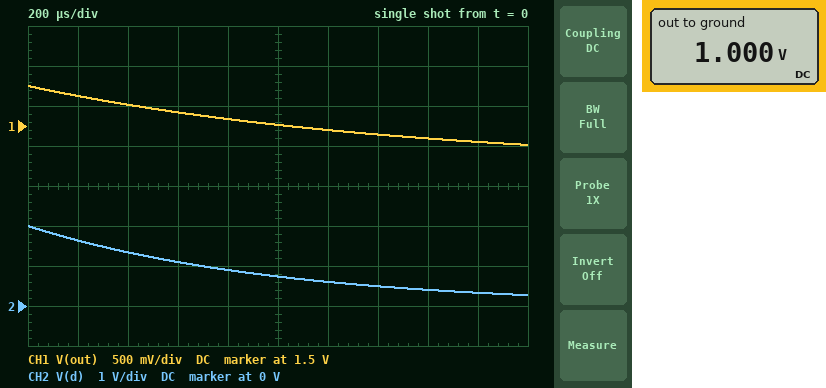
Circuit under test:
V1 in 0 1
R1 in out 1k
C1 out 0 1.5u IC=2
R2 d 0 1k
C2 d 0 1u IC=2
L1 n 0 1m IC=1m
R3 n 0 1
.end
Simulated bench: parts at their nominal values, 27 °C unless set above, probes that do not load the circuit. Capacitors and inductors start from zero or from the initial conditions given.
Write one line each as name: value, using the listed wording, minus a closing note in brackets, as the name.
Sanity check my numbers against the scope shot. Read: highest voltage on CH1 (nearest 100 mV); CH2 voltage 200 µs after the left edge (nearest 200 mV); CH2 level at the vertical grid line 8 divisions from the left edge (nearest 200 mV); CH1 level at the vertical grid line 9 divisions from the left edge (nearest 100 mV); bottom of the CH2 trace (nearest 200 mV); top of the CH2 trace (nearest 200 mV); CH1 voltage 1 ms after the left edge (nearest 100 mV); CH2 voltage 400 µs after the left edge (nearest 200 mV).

highest voltage on CH1: 2.0 V
CH2 voltage 200 µs after the left edge: 1.6 V
CH2 level at the vertical grid line 8 divisions from the left edge: 400 mV
CH1 level at the vertical grid line 9 divisions from the left edge: 1.3 V
bottom of the CH2 trace: 200 mV
top of the CH2 trace: 2.0 V
CH1 voltage 1 ms after the left edge: 1.5 V
CH2 voltage 400 µs after the left edge: 1.4 V
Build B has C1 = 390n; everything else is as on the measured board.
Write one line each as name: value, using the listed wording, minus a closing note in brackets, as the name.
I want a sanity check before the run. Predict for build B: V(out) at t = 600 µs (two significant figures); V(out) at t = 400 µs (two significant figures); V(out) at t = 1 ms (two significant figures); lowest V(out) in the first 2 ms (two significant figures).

V(out) at t = 600 µs: 1.2 V
V(out) at t = 400 µs: 1.4 V
V(out) at t = 1 ms: 1.1 V
lowest V(out) in the first 2 ms: 1.0 V
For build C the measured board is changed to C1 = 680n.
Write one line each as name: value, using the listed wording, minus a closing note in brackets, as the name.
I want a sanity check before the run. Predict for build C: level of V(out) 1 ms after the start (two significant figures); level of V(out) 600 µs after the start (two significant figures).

level of V(out) 1 ms after the start: 1.2 V
level of V(out) 600 µs after the start: 1.4 V
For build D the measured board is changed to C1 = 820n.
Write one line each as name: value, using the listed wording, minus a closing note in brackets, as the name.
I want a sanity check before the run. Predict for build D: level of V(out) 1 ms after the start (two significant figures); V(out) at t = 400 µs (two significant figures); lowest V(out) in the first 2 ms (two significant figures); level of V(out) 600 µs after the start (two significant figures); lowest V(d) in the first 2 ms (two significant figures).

level of V(out) 1 ms after the start: 1.3 V
V(out) at t = 400 µs: 1.6 V
lowest V(out) in the first 2 ms: 1.1 V
level of V(out) 600 µs after the start: 1.5 V
lowest V(d) in the first 2 ms: 270 mV
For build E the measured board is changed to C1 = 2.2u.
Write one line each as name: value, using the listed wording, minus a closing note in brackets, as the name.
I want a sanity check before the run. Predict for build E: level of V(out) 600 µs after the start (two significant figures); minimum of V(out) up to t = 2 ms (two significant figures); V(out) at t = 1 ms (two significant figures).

level of V(out) 600 µs after the start: 1.8 V
minimum of V(out) up to t = 2 ms: 1.4 V
V(out) at t = 1 ms: 1.6 V
